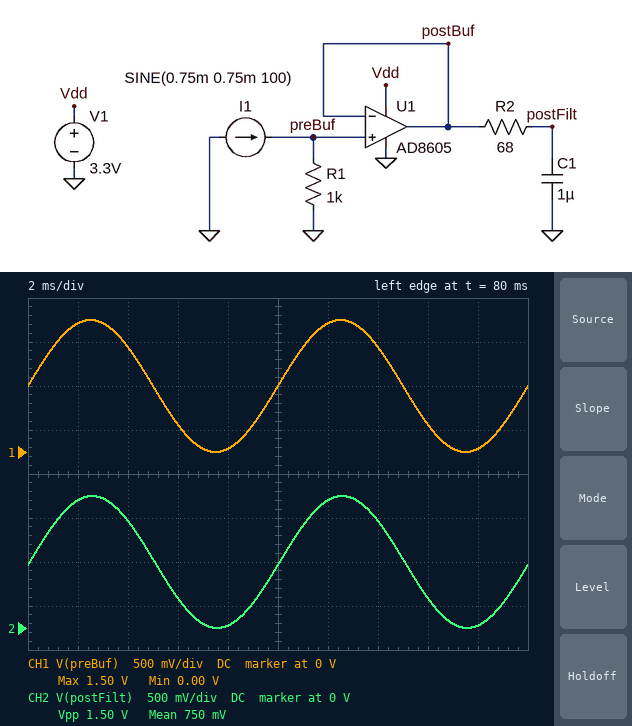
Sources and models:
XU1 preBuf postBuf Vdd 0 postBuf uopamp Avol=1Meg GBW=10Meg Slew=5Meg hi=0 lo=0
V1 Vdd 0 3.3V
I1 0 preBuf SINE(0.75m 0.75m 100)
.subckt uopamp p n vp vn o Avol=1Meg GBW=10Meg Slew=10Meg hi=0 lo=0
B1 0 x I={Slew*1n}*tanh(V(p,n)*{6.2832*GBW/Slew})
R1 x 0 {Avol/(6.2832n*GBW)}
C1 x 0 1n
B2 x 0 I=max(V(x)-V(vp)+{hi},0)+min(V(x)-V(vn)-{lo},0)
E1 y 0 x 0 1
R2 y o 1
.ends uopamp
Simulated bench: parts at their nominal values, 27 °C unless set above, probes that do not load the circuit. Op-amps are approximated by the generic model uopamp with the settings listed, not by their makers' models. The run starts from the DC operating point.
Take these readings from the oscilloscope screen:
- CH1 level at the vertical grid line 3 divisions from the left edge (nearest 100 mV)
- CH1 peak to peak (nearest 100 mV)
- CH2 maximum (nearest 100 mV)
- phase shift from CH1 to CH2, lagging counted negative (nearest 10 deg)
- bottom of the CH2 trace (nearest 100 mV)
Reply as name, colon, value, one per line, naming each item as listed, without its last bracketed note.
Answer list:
CH1 level at the vertical grid line 3 divisions from the left edge: 300 mV
CH1 peak to peak: 1.5 V
CH2 maximum: 1.5 V
phase shift from CH1 to CH2, lagging counted negative: 0 deg
bottom of the CH2 trace: 0 V
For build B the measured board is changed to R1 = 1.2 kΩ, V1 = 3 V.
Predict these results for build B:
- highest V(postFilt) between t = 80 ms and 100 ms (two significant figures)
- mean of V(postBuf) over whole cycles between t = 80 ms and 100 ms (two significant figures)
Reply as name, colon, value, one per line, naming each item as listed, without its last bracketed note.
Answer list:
highest V(postFilt) between t = 80 ms and 100 ms: 1.8 V
mean of V(postBuf) over whole cycles between t = 80 ms and 100 ms: 900 mV
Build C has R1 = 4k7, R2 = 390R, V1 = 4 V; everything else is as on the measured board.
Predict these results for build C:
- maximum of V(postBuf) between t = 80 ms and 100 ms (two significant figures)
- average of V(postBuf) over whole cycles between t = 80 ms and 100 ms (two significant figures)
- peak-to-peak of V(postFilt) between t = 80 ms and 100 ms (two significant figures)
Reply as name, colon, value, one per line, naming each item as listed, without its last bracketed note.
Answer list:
maximum of V(postBuf) between t = 80 ms and 100 ms: 4.0 V
average of V(postBuf) over whole cycles between t = 80 ms and 100 ms: 2.6 V
peak-to-peak of V(postFilt) between t = 80 ms and 100 ms: 3.9 V
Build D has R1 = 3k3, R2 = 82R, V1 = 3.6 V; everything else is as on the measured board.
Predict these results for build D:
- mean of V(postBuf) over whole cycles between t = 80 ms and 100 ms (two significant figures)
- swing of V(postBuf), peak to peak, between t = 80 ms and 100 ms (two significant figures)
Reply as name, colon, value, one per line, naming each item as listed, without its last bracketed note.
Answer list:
mean of V(postBuf) over whole cycles between t = 80 ms and 100 ms: 2.2 V
swing of V(postBuf), peak to peak, between t = 80 ms and 100 ms: 3.6 V
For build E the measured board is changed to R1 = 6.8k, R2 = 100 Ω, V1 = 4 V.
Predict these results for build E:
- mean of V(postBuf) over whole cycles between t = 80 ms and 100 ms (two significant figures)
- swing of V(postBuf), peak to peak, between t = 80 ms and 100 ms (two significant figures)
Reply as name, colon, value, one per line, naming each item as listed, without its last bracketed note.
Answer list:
mean of V(postBuf) over whole cycles between t = 80 ms and 100 ms: 2.9 V
swing of V(postBuf), peak to peak, between t = 80 ms and 100 ms: 4.0 V
